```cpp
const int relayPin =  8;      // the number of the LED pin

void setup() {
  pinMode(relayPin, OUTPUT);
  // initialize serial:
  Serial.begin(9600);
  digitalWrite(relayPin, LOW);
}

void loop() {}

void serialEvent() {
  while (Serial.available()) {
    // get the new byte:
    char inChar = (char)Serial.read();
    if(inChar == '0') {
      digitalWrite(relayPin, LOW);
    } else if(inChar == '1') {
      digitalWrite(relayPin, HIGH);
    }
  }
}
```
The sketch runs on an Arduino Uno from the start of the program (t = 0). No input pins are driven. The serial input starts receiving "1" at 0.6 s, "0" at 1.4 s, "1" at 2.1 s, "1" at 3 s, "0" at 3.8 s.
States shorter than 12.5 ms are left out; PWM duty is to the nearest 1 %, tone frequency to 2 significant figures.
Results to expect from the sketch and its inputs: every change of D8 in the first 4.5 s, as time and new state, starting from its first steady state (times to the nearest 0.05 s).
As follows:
0 s low; 0.6 s high; 1.4 s low; 2.1 s high; 3.8 s low
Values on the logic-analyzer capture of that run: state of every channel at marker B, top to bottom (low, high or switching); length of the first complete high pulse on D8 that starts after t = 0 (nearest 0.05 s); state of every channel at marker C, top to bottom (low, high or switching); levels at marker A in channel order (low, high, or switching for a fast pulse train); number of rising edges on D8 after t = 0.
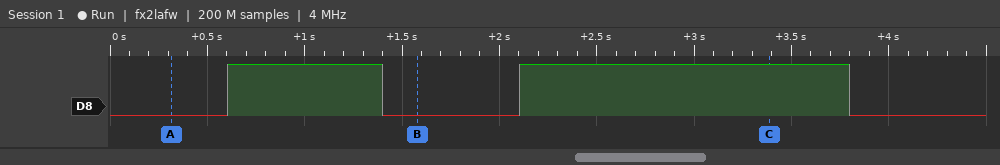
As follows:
D8 low
0.80 s
D8 high
D8 low
2
